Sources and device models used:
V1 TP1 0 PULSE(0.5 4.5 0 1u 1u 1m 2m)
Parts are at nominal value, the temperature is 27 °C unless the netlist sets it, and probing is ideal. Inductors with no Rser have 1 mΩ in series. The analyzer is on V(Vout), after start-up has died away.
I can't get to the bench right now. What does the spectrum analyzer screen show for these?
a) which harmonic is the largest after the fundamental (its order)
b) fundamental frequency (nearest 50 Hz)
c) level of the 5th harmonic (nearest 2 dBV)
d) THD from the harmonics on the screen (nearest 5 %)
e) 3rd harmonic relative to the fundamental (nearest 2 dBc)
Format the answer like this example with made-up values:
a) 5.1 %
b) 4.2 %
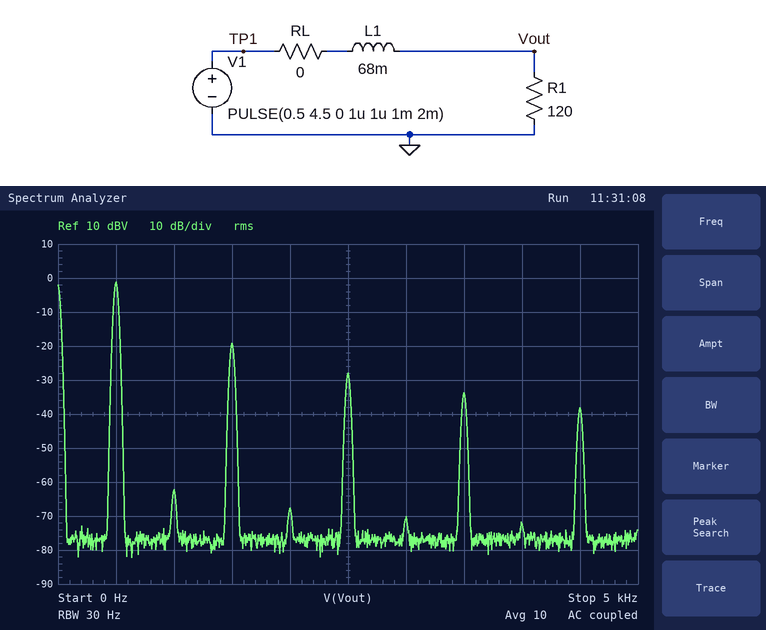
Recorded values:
a) 3
b) 500 Hz
c) -28 dBV
d) 15 %
e) -18 dBc
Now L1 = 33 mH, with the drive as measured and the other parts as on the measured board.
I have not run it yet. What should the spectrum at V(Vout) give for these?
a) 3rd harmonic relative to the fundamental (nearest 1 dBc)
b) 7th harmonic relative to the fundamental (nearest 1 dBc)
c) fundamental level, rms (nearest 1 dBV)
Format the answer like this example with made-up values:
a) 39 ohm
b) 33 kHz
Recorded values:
a) -16 dBc
b) -30 dBc
c) 3 dBV
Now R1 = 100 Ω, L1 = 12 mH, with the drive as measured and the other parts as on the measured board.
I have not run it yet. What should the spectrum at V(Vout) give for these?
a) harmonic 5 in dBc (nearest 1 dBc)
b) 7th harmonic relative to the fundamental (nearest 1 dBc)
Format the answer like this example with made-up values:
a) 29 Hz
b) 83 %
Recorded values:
a) -20 dBc
b) -25 dBc
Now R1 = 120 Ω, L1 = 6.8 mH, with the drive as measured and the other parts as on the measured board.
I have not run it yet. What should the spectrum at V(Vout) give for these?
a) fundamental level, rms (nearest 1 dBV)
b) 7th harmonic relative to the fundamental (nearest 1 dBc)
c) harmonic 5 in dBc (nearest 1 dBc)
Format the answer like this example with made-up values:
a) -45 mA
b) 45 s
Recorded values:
a) 5 dBV
b) -21 dBc
c) -16 dBc
